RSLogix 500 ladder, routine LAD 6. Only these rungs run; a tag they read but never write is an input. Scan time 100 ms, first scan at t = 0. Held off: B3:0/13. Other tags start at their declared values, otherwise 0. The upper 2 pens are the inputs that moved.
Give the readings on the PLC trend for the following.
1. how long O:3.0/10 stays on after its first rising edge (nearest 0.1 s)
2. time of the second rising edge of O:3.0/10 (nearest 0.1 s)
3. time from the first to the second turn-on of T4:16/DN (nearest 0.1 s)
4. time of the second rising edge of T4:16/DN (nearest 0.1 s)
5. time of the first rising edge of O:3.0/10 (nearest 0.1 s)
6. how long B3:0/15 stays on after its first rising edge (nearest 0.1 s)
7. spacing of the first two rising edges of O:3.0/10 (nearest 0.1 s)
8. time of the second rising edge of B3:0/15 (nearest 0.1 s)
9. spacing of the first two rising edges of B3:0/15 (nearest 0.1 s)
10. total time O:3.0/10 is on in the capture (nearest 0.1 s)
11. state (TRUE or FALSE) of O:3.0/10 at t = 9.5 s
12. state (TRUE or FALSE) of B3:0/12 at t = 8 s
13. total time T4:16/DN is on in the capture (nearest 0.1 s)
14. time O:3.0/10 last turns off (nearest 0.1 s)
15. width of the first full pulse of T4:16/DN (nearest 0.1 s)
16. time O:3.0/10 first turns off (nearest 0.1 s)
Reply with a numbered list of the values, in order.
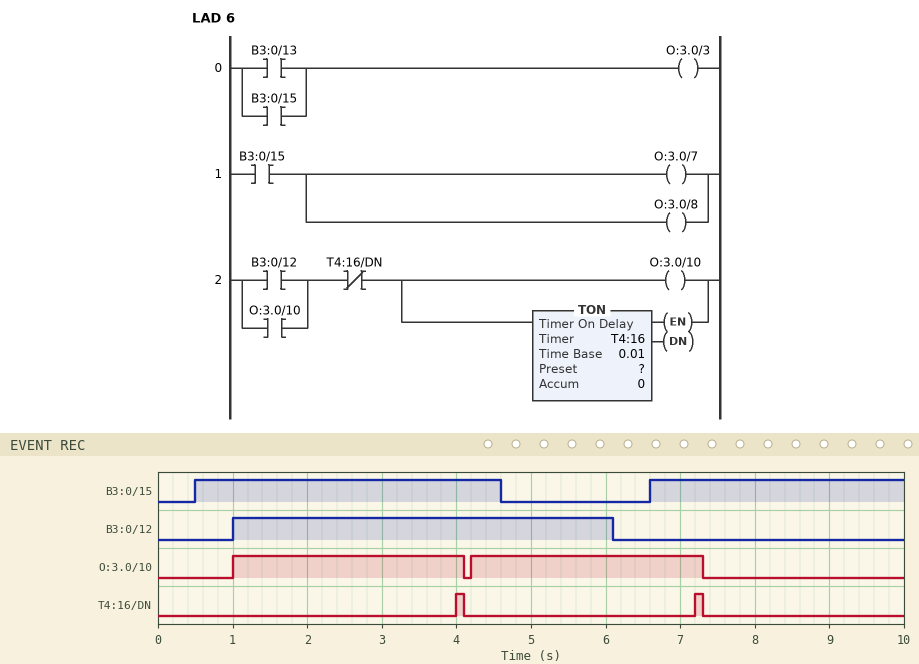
1. 3.1 s
2. 4.2 s
3. 3.2 s
4. 7.2 s
5. 1.0 s
6. 4.1 s
7. 3.2 s
8. 6.6 s
9. 6.1 s
10. 6.2 s
11. FALSE
12. FALSE
13. 0.2 s
14. 7.3 s
15. 0.1 s
16. 4.1 s
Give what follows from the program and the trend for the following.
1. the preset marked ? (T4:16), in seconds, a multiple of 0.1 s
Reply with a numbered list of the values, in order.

1. 3.0 s
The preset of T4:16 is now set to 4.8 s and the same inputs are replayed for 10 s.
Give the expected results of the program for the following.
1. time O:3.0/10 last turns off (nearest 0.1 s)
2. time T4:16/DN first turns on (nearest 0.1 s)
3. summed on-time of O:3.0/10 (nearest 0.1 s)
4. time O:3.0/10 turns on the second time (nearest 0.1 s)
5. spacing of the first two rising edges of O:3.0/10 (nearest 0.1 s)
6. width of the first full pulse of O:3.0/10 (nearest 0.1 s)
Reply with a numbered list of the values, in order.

1. 5.9 s
2. 5.8 s
3. 8.9 s
4. 6.0 s
5. 5.0 s
6. 4.9 s
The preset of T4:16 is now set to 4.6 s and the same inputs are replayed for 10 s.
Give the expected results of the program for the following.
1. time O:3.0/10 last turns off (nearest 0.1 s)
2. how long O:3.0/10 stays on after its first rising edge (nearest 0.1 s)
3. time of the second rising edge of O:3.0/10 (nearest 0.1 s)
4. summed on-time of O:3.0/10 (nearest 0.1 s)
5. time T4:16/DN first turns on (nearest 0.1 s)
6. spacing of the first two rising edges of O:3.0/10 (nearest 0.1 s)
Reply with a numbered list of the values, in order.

1. 5.7 s
2. 4.7 s
3. 5.8 s
4. 8.9 s
5. 5.6 s
6. 4.8 s
